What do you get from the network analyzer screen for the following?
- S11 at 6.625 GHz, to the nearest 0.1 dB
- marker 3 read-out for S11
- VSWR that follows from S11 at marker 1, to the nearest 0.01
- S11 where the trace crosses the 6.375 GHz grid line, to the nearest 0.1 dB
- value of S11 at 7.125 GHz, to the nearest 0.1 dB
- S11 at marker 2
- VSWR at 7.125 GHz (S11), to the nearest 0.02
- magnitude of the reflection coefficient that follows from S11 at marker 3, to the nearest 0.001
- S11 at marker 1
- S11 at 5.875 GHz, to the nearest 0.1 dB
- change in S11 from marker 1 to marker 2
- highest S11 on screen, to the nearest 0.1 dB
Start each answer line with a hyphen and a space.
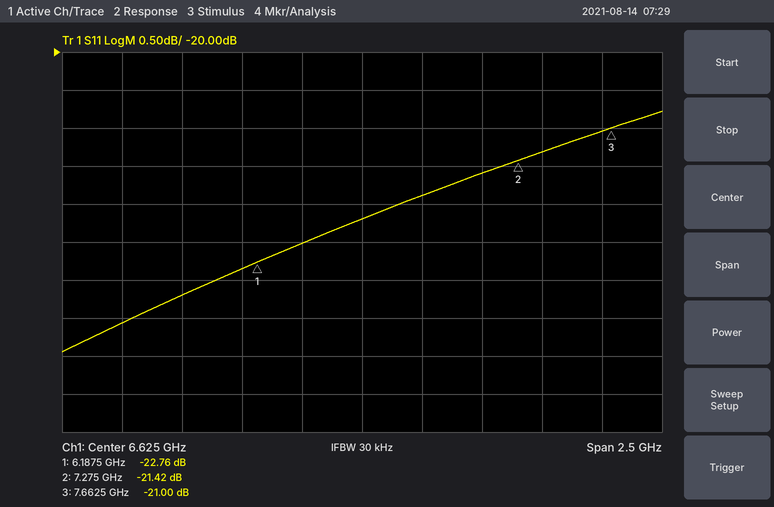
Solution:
- -22.2 dB
- -21.00 dB
- 1.16
- -22.5 dB
- -21.6 dB
- -21.42 dB
- 1.18
- 0.089
- -22.76 dB
- -23.2 dB
- 1.34 dB
- -20.8 dB
